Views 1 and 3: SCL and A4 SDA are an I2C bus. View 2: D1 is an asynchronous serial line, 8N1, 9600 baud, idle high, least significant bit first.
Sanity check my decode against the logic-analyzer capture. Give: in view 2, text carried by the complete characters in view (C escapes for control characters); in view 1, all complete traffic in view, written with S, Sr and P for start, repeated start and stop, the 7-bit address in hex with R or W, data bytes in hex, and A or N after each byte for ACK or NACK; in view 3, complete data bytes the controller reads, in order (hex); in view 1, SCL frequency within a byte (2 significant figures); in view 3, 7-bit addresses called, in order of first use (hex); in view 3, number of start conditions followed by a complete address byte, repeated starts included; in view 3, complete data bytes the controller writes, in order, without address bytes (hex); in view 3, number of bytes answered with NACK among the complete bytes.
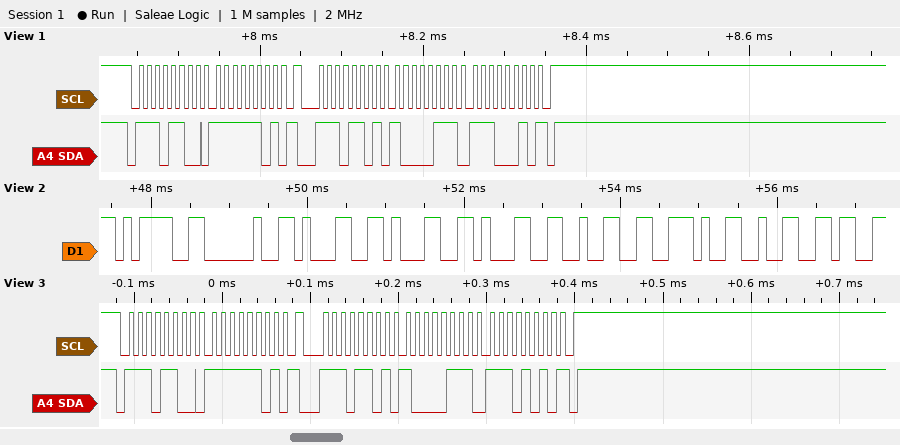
"= 1112.2"
S 76W A FD A Sr 76R A 87 A E2 N P
87 EA
100 kHz
0x76
2
FD
1
